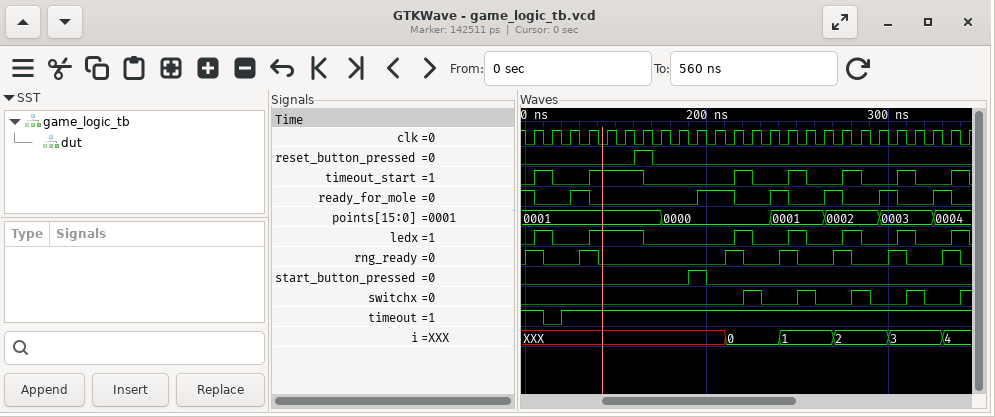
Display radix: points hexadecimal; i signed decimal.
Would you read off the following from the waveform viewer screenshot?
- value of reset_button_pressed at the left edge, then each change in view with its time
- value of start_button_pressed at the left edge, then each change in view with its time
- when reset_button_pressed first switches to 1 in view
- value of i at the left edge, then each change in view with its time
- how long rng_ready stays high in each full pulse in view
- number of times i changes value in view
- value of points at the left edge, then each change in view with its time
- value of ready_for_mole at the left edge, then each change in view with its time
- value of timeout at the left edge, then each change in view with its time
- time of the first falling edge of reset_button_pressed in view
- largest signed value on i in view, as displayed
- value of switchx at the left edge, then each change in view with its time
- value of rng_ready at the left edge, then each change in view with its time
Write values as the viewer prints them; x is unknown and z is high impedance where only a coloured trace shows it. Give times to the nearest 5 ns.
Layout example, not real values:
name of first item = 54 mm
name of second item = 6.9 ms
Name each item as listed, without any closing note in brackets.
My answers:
value of reset_button_pressed at the left edge, then each change in view with its time = 0, 1 at 160 ns, 0 at 170 ns
value of start_button_pressed at the left edge, then each change in view with its time = 0, 1 at 190 ns, 0 at 200 ns
when reset_button_pressed first switches to 1 in view = 160 ns
value of i at the left edge, then each change in view with its time = XXX, 0 at 210 ns, 1 at 240 ns, 2 at 270 ns, 3 at 300 ns, 4 at 330 ns
how long rng_ready stays high in each full pulse in view = 10 ns, 10 ns, 10 ns, 10 ns, 10 ns, 10 ns, 10 ns
number of times i changes value in view = 5
value of points at the left edge, then each change in view with its time = 0001, 0000 at 175 ns, 0001 at 235 ns, 0002 at 265 ns, 0003 at 295 ns, 0004 at 325 ns
value of ready_for_mole at the left edge, then each change in view with its time = 1, 0 at 105 ns, 1 at 125 ns, 0 at 135 ns, 1 at 195 ns, 0 at 215 ns, 1 at 235 ns, 0 at 245 ns, 1 at 265 ns, 0 at 275 ns, 1 at 295 ns, 0 at 305 ns, 1 at 325 ns, 0 at 335 ns
value of timeout at the left edge, then each change in view with its time = 1, 0 at 110 ns, 1 at 120 ns
time of the first falling edge of reset_button_pressed in view = 170 ns
largest signed value on i in view, as displayed = 4
value of switchx at the left edge, then each change in view with its time = 0, 1 at 220 ns, 0 at 230 ns, 1 at 250 ns, 0 at 260 ns, 1 at 280 ns, 0 at 290 ns, 1 at 310 ns, 0 at 320 ns, 1 at 340 ns
value of rng_ready at the left edge, then each change in view with its time = 0, 1 at 100 ns, 0 at 110 ns, 1 at 130 ns, 0 at 140 ns, 1 at 210 ns, 0 at 220 ns, 1 at 240 ns, 0 at 250 ns, 1 at 270 ns, 0 at 280 ns, 1 at 300 ns, 0 at 310 ns, 1 at 330 ns, 0 at 340 ns
